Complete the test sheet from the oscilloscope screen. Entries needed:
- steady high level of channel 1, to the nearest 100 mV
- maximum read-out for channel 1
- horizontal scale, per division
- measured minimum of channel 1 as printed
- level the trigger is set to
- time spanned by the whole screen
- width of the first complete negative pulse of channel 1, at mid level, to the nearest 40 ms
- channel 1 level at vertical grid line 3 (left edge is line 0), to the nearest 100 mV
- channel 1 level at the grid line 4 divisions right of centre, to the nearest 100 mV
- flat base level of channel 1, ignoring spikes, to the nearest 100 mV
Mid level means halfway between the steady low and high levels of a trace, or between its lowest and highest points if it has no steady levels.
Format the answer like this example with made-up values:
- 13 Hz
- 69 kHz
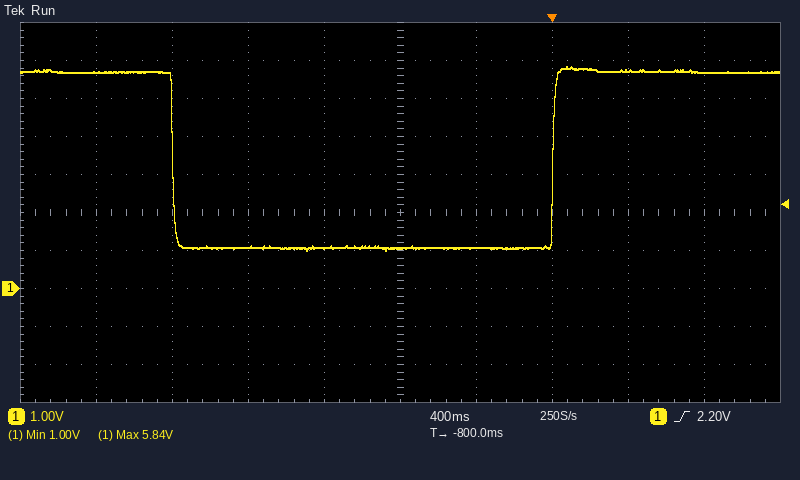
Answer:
- 5.7 V
- 5.84 V
- 400 ms
- 1.00 V
- 2.20 V
- 4 s
- 2.00 s
- 1.1 V
- 5.7 V
- 1.1 V
